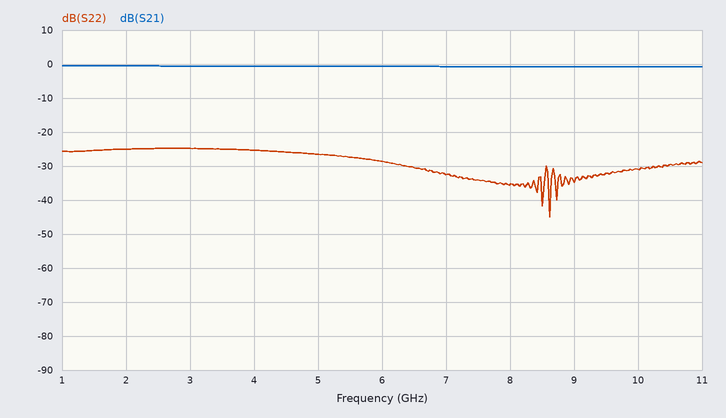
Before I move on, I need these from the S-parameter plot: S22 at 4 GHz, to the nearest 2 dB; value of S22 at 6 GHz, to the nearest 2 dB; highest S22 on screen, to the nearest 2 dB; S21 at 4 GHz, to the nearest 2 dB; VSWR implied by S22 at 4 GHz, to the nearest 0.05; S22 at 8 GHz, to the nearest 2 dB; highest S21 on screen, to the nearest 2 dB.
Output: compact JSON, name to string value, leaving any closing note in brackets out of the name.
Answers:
{"S22 at 4 GHz, to the nearest 2 dB": "-26 dB", "value of S22 at 6 GHz, to the nearest 2 dB": "-28 dB", "highest S22 on screen, to the nearest 2 dB": "-24 dB", "S21 at 4 GHz, to the nearest 2 dB": "0 dB", "VSWR implied by S22 at 4 GHz, to the nearest 0.05": "1.10", "S22 at 8 GHz, to the nearest 2 dB": "-36 dB", "highest S21 on screen, to the nearest 2 dB": "0 dB"}
